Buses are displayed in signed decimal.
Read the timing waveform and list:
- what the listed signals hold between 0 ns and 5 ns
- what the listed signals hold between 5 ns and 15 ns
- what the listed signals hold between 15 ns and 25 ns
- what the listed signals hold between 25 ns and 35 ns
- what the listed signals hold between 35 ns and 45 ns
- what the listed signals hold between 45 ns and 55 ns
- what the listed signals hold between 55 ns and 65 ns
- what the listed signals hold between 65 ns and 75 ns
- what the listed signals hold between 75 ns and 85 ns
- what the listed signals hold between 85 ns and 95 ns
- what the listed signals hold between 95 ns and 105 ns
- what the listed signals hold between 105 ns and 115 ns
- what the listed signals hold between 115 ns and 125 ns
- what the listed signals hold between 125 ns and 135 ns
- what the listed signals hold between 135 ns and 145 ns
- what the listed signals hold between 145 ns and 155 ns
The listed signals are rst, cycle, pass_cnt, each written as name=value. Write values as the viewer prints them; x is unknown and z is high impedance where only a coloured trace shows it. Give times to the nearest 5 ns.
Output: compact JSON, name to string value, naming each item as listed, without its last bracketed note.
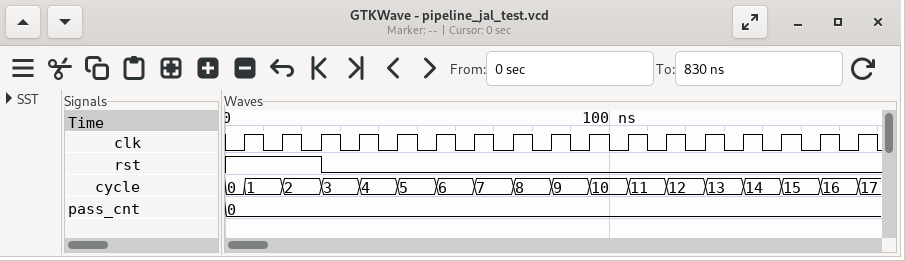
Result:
{"what the listed signals hold between 0 ns and 5 ns": "rst=1, cycle=0, pass_cnt=0", "what the listed signals hold between 5 ns and 15 ns": "rst=1, cycle=1, pass_cnt=0", "what the listed signals hold between 15 ns and 25 ns": "rst=1, cycle=2, pass_cnt=0", "what the listed signals hold between 25 ns and 35 ns": "rst=0, cycle=3, pass_cnt=0", "what the listed signals hold between 35 ns and 45 ns": "rst=0, cycle=4, pass_cnt=0", "what the listed signals hold between 45 ns and 55 ns": "rst=0, cycle=5, pass_cnt=0", "what the listed signals hold between 55 ns and 65 ns": "rst=0, cycle=6, pass_cnt=0", "what the listed signals hold between 65 ns and 75 ns": "rst=0, cycle=7, pass_cnt=0", "what the listed signals hold between 75 ns and 85 ns": "rst=0, cycle=8, pass_cnt=0", "what the listed signals hold between 85 ns and 95 ns": "rst=0, cycle=9, pass_cnt=0", "what the listed signals hold between 95 ns and 105 ns": "rst=0, cycle=10, pass_cnt=0", "what the listed signals hold between 105 ns and 115 ns": "rst=0, cycle=11, pass_cnt=0", "what the listed signals hold between 115 ns and 125 ns": "rst=0, cycle=12, pass_cnt=0", "what the listed signals hold between 125 ns and 135 ns": "rst=0, cycle=13, pass_cnt=0", "what the listed signals hold between 135 ns and 145 ns": "rst=0, cycle=14, pass_cnt=0", "what the listed signals hold between 145 ns and 155 ns": "rst=0, cycle=15, pass_cnt=0"}
